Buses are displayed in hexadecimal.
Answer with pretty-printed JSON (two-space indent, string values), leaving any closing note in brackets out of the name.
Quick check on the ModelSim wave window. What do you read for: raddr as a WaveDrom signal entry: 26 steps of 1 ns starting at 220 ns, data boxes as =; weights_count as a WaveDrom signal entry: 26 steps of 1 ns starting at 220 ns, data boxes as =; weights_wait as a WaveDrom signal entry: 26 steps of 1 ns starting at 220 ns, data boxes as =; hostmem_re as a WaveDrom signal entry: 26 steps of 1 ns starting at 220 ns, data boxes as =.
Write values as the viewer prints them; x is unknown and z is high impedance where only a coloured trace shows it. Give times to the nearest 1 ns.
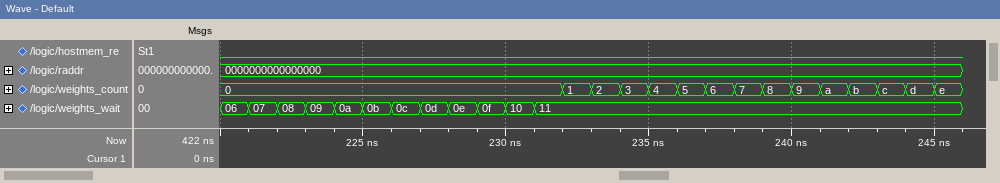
{
  "raddr as a WaveDrom signal entry: 26 steps of 1 ns starting at 220 ns, data boxes as =": "{name: 'raddr', wave: '=.........................', data: '0000000000000000'}",
  "weights_count as a WaveDrom signal entry: 26 steps of 1 ns starting at 220 ns, data boxes as =": "{name: 'weights_count', wave: '=...........==============', data: '0 1 2 3 4 5 6 7 8 9 a b c d e'}",
  "weights_wait as a WaveDrom signal entry: 26 steps of 1 ns starting at 220 ns, data boxes as =": "{name: 'weights_wait', wave: '============..............', data: '06 07 08 09 0a 0b 0c 0d 0e 0f 10 11'}",
  "hostmem_re as a WaveDrom signal entry: 26 steps of 1 ns starting at 220 ns, data boxes as =": "{name: 'hostmem_re', wave: '0.........................'}"
}
